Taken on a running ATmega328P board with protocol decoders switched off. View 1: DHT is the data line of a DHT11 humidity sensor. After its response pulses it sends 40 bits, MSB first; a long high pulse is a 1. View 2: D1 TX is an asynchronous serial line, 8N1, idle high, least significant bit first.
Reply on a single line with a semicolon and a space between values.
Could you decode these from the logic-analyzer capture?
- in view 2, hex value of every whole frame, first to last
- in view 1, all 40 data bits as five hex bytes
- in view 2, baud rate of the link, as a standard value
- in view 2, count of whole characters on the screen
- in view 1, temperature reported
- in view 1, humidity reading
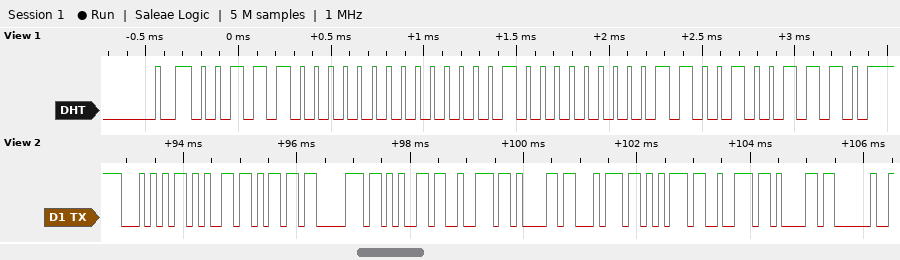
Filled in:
54 65 6D 70 65 72 61 74 75 72 61 20; 38 00 10 06 4E; 9600 baud; 12; 16.6 °C; 56 %
